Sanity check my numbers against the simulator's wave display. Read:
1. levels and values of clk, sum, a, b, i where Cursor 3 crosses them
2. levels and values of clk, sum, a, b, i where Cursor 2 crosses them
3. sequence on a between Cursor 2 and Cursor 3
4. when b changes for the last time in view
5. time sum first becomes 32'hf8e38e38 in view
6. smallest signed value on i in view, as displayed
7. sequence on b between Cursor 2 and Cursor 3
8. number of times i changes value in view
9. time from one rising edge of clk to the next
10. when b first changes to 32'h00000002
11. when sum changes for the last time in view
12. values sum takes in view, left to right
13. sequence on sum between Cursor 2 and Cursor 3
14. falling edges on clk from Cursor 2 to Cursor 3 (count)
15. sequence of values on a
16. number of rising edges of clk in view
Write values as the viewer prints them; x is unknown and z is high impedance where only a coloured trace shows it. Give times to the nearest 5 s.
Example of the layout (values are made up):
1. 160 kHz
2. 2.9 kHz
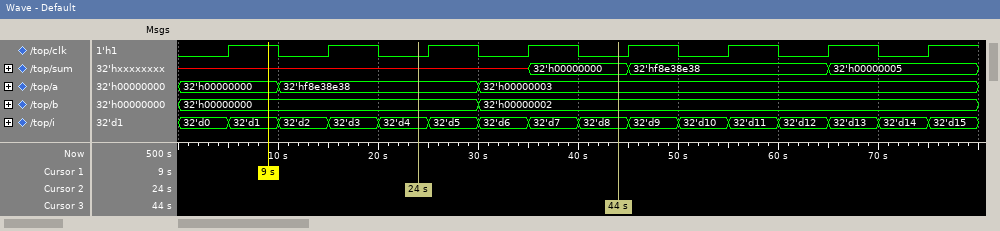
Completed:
1. clk=0, sum=32'h00000000, a=32'h00000003, b=32'h00000002, i=32'd8
2. clk=0, sum=x, a=32'hf8e38e38, b=32'h00000000, i=32'd4
3. 32'hf8e38e38, 32'h00000003
4. 30 s
5. 45 s
6. 32'd0
7. 32'h00000000, 32'h00000002
8. 15
9. 10 s
10. 30 s
11. 65 s
12. x, 32'h00000000, 32'hf8e38e38, 32'h00000005
13. x, 32'h00000000
14. 2
15. 32'h00000000, 32'hf8e38e38, 32'h00000003
16. 8
